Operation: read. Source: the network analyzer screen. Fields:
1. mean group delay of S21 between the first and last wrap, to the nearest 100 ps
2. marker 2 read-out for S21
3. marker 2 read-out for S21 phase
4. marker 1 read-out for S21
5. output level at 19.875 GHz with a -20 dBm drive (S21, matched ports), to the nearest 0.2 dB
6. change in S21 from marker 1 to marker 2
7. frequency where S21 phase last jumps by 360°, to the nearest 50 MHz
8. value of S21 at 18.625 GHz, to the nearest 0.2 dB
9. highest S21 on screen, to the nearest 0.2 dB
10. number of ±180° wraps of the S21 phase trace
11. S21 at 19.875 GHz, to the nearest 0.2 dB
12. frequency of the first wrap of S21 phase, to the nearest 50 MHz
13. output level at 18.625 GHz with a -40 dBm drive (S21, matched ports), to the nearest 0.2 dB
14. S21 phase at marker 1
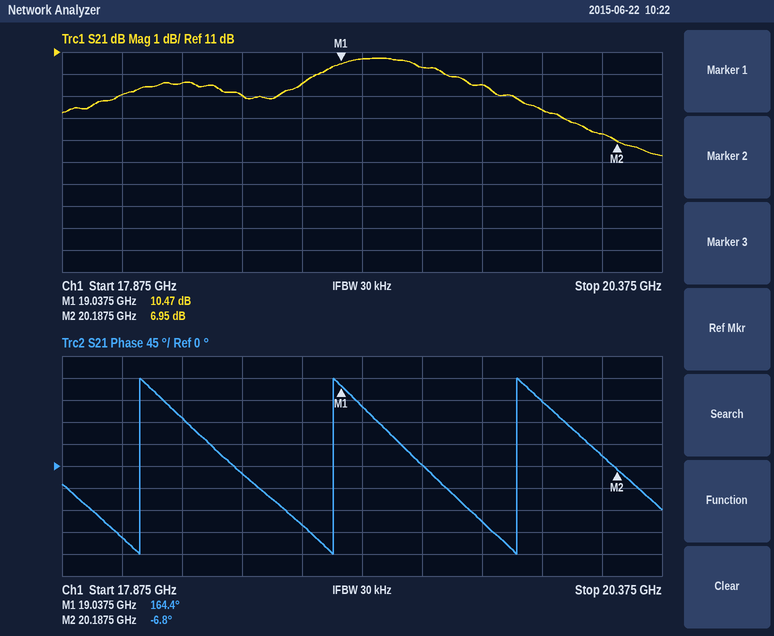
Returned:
1.3 ns
6.95 dB
-6.8°
10.47 dB
-11.6 dBm
-3.52 dB
19.75 GHz
9.0 dB
10.8 dB
3
8.4 dB
18.20 GHz
-31.0 dBm
164.4°
